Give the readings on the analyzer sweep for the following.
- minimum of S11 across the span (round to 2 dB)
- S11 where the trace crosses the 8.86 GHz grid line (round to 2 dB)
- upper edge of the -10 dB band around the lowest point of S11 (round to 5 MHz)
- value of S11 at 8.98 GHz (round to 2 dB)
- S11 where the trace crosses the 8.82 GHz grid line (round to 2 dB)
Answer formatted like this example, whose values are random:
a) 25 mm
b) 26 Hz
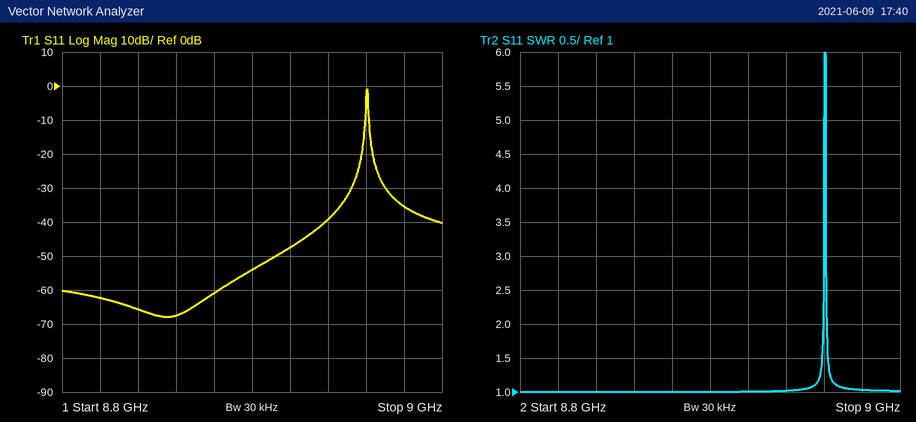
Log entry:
a) -68 dB
b) -68 dB
c) 8.960 GHz
d) -36 dB
e) -62 dB
